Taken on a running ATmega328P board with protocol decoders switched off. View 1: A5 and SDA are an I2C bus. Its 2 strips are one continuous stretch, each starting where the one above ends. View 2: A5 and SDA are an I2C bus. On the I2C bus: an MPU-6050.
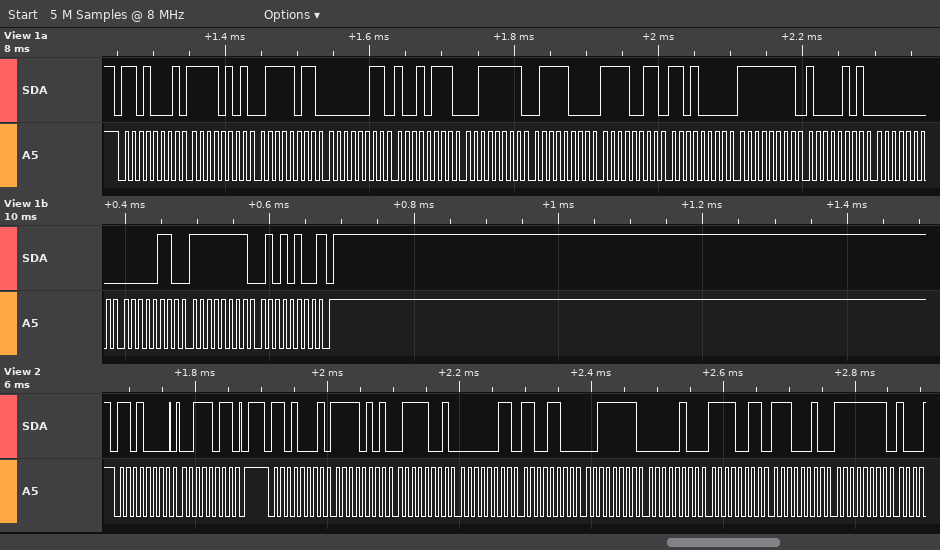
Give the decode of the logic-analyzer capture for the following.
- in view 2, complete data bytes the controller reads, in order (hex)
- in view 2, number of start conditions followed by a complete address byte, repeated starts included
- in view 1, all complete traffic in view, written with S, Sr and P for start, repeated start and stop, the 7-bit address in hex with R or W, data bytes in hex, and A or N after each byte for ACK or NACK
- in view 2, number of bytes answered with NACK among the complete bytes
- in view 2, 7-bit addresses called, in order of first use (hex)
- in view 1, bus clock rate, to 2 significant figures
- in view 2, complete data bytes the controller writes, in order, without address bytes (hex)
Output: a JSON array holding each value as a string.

["F5 79 03 CC 3F 04 F3 E2 FF", "2", "S 68R A F5 A 7B A 03 A 97 A 3F A 78 A F3 A D0 A FF A 85 A 00 A 06 A FF A 54 N P", "0", "0x68", "100 kHz", "3B"]
